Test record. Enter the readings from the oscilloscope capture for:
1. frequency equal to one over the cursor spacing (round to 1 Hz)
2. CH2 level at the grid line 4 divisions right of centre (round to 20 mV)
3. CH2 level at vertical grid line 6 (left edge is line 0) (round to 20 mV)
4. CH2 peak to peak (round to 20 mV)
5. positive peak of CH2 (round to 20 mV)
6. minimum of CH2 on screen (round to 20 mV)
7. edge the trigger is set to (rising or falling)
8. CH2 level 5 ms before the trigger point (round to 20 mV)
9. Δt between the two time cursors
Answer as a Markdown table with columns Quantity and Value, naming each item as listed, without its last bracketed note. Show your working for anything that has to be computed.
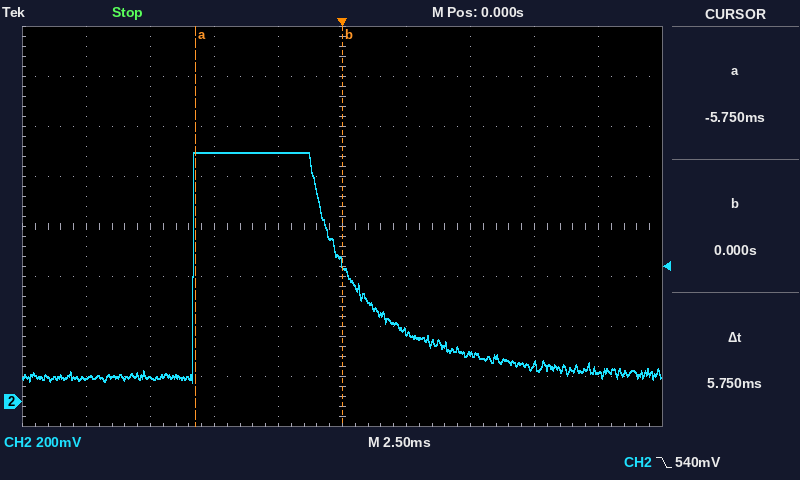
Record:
| Quantity | Value |
|---|---|
| frequency equal to one over the cursor spacing | 1 / 5.75 ms ≈ 174 Hz |
| CH2 level at the grid line 4 divisions right of centre | 120 mV |
| CH2 level at vertical grid line 6 (left edge is line 0) | 280 mV |
| CH2 peak to peak | 1.00 V − (80 mV) = 920 mV |
| positive peak of CH2 | 1.00 V |
| minimum of CH2 on screen | 80 mV |
| edge the trigger is set to | falling |
| CH2 level 5 ms before the trigger point | 1.00 V |
| Δt between the two time cursors | 5.75 ms |
